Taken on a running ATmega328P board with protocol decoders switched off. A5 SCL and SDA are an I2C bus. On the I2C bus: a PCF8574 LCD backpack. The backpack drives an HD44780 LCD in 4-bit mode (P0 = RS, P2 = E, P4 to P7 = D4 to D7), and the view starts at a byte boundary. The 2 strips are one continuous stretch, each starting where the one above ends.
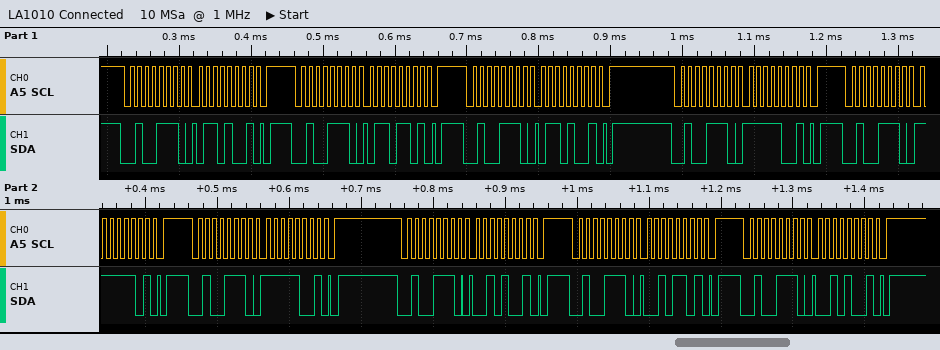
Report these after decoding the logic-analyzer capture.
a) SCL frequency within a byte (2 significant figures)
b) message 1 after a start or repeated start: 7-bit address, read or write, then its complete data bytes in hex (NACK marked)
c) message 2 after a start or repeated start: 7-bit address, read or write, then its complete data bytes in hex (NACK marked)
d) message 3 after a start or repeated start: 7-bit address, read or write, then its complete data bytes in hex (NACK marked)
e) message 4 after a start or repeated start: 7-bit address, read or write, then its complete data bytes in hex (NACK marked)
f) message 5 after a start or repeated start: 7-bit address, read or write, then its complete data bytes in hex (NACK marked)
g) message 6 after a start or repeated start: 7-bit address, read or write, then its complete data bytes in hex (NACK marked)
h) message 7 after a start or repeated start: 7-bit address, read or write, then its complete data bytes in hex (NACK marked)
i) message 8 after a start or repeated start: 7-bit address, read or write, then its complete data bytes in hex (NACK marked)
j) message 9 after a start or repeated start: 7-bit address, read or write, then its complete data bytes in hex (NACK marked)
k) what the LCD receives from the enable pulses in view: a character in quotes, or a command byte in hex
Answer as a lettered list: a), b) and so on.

a) 100 kHz
b) 0x27 write: 69
c) 0x27 write: 6D
d) 0x27 write: 69
e) 0x27 write: F9
f) 0x27 write: FD
g) 0x27 write: F9
h) 0x27 write: 29
i) 0x27 write: 2D
j) 0x27 write: 29
k) 'o'
